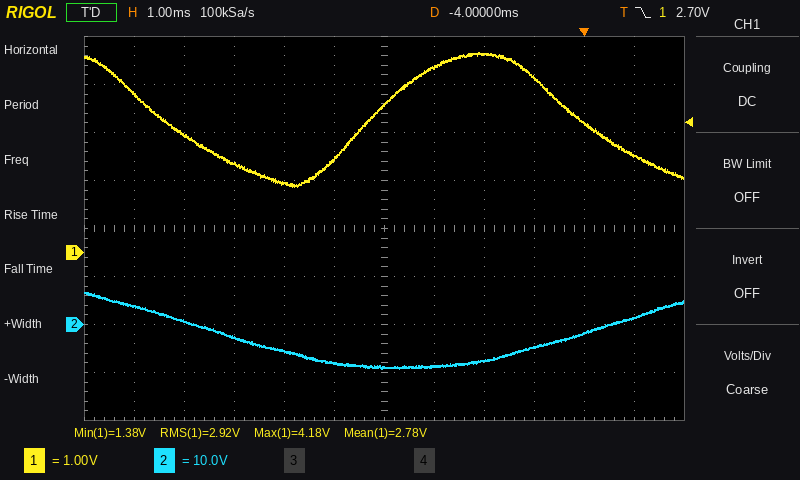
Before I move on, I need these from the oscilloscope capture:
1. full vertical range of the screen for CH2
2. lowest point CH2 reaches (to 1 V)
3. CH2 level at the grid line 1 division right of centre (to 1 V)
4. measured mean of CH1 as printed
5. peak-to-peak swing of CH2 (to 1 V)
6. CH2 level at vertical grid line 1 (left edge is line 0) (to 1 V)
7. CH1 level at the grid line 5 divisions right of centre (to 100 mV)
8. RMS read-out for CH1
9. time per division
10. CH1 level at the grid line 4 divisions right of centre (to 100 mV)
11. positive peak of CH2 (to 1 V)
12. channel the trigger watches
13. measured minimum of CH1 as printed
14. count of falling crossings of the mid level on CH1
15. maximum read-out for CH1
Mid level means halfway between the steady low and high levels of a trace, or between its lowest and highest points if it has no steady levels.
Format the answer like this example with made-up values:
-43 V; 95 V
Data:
80 V; -9 V; -9 V; 2.78 V; 16 V; 4 V; 2.0 V; 2.92 V; 1 ms; 2.7 V; 7 V; CH1; 1.38 V; 2; 4.18 V
